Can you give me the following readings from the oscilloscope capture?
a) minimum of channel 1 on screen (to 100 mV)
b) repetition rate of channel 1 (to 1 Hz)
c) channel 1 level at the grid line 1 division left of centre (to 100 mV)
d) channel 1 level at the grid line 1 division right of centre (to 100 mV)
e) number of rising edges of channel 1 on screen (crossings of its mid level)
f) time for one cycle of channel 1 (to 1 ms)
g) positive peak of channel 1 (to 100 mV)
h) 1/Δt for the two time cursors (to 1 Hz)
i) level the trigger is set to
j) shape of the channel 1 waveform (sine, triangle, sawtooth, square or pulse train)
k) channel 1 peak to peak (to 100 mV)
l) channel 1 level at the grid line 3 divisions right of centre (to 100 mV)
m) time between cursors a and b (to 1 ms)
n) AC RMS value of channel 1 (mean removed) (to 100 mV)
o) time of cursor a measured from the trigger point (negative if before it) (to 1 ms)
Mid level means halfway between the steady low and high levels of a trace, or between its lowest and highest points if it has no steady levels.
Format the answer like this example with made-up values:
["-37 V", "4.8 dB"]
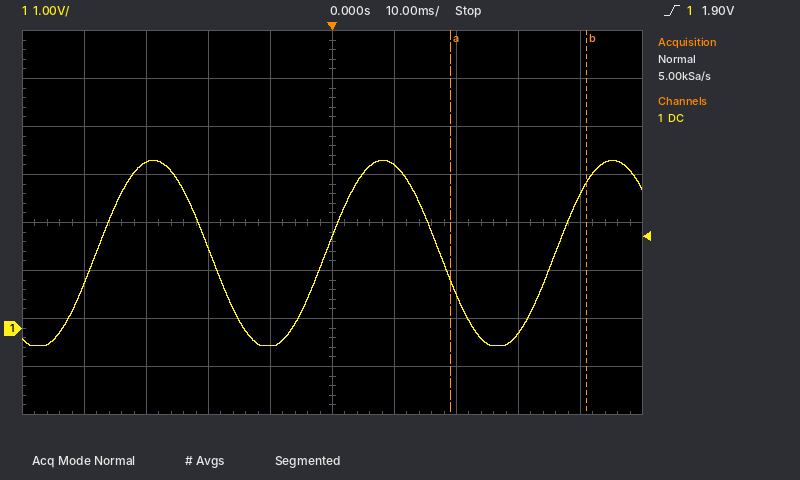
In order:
["-400 mV", "27 Hz", "-400 mV", "3.4 V", "3", "37 ms", "3.5 V", "45 Hz", "1.90 V", "sine", "3.9 V", "-100 mV", "22 ms", "1.4 V", "+19 ms"]
